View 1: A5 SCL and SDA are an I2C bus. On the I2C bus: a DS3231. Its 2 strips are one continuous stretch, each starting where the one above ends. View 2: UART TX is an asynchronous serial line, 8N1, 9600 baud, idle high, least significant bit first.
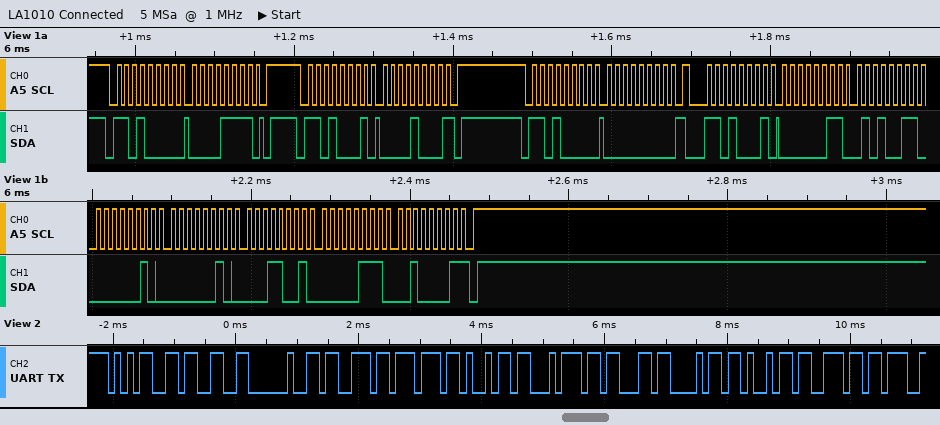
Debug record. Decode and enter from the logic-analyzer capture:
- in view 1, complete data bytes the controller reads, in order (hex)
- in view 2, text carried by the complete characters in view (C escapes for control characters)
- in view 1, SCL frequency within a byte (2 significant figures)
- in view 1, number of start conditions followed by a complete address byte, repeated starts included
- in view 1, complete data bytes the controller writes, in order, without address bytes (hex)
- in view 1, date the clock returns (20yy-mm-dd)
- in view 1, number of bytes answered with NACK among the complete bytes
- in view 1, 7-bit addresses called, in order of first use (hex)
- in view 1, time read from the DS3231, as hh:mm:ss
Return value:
08 03 53 02 02 19 07 21
"53 switchin"
100 kHz
4
0F 00
2021-07-19
2
0x68
02:53:03
